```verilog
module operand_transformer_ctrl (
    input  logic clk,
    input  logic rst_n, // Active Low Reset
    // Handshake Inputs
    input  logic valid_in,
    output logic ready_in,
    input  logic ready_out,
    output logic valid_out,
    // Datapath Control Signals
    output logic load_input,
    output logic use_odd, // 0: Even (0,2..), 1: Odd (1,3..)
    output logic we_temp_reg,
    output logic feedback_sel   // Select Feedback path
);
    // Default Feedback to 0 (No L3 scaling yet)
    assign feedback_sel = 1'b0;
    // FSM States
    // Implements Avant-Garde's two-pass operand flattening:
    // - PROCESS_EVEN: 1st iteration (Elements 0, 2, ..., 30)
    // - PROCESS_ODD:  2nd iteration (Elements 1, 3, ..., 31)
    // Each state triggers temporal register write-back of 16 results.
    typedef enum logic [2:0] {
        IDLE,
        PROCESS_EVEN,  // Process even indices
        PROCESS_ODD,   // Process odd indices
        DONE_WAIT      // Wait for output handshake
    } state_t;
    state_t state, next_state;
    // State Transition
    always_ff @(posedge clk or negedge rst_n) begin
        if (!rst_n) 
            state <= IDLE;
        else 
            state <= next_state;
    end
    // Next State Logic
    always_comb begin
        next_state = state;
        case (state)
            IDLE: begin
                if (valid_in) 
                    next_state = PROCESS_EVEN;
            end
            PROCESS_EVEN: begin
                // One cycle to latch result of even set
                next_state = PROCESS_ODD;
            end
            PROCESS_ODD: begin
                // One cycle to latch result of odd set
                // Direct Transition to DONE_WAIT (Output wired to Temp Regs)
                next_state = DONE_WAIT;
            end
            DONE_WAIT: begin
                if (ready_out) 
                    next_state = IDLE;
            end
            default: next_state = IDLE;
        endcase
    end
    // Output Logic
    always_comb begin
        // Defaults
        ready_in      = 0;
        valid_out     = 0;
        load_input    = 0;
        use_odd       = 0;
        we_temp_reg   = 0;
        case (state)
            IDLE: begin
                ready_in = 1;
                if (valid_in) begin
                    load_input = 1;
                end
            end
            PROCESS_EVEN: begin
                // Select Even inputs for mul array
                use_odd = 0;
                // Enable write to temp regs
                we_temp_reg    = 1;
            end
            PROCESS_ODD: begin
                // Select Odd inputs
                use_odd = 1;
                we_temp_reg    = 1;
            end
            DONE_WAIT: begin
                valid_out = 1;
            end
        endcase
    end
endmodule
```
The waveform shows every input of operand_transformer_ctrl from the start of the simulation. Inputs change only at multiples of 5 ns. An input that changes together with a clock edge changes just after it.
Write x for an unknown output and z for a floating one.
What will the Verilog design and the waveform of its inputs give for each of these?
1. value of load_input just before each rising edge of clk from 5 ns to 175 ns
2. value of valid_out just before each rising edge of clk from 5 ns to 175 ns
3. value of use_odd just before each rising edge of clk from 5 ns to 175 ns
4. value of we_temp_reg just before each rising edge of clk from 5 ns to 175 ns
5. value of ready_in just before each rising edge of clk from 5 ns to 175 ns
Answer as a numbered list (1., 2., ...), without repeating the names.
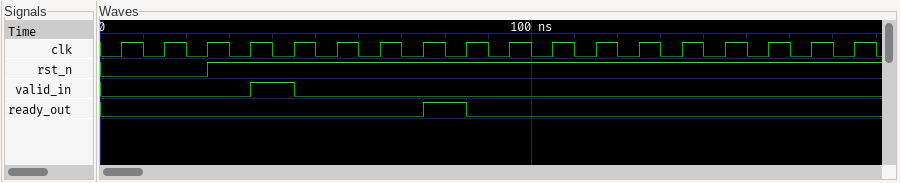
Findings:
1. 0 0 0 0 1 0 0 0 0 0 0 0 0 0 0 0 0 0
2. 0 0 0 0 0 0 0 1 1 0 0 0 0 0 0 0 0 0
3. 0 0 0 0 0 0 1 0 0 0 0 0 0 0 0 0 0 0
4. 0 0 0 0 0 1 1 0 0 0 0 0 0 0 0 0 0 0
5. 1 1 1 1 1 0 0 0 0 1 1 1 1 1 1 1 1 1
